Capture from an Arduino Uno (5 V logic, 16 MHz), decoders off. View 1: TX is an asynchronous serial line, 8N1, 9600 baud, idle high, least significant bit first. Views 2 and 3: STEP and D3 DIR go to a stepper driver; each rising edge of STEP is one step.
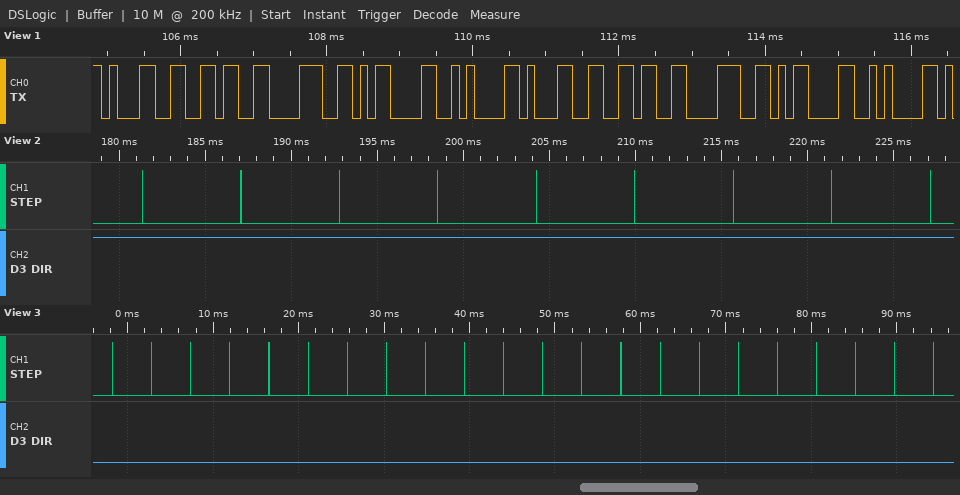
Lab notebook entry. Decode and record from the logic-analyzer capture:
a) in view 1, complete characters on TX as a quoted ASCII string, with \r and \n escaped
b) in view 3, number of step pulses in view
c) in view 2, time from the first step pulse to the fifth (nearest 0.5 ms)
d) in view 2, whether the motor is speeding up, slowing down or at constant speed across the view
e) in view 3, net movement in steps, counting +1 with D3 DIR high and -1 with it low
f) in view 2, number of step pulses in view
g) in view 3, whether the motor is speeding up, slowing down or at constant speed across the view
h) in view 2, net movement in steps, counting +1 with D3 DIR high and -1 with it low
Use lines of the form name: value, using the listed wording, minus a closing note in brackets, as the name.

in view 1, complete characters on TX as a quoted ASCII string, with \r and \n escaped: "168\r\n168\r\n"
in view 3, number of step pulses in view: 22
in view 2, time from the first step pulse to the fifth: 23.0 ms
in view 2, whether the motor is speeding up, slowing down or at constant speed across the view: constant speed
in view 3, net movement in steps, counting +1 with D3 DIR high and -1 with it low: -22
in view 2, number of step pulses in view: 9
in view 3, whether the motor is speeding up, slowing down or at constant speed across the view: constant speed
in view 2, net movement in steps, counting +1 with D3 DIR high and -1 with it low: +9
